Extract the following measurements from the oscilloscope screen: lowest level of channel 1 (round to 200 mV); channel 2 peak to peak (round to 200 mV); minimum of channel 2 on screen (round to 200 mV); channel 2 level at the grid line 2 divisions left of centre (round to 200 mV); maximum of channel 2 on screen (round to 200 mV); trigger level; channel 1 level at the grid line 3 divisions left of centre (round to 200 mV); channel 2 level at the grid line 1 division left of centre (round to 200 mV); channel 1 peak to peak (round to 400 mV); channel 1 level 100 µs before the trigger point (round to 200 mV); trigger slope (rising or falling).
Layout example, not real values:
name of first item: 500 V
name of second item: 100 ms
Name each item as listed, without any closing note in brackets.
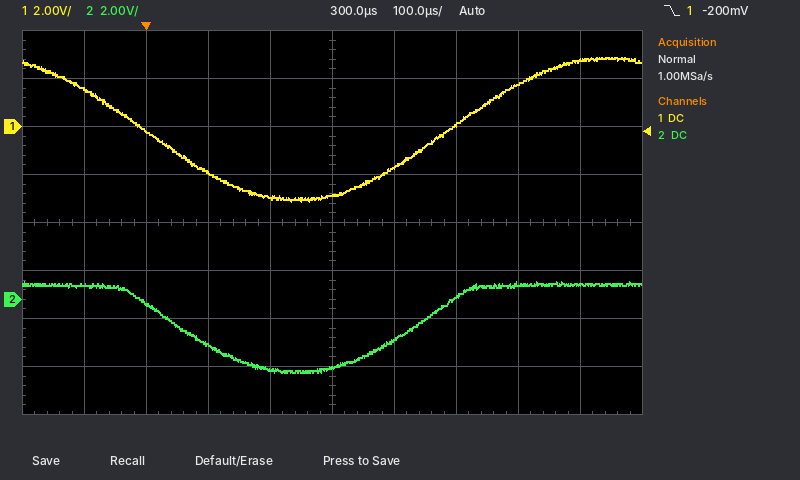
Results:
lowest level of channel 1: -3.2 V
channel 2 peak to peak: 3.8 V
minimum of channel 2 on screen: -3.0 V
channel 2 level at the grid line 2 divisions left of centre: -1.8 V
maximum of channel 2 on screen: 800 mV
trigger level: -200 mV
channel 1 level at the grid line 3 divisions left of centre: -200 mV
channel 2 level at the grid line 1 division left of centre: -3.0 V
channel 1 peak to peak: 6.0 V
channel 1 level 100 µs before the trigger point: 1.6 V
trigger slope: falling
